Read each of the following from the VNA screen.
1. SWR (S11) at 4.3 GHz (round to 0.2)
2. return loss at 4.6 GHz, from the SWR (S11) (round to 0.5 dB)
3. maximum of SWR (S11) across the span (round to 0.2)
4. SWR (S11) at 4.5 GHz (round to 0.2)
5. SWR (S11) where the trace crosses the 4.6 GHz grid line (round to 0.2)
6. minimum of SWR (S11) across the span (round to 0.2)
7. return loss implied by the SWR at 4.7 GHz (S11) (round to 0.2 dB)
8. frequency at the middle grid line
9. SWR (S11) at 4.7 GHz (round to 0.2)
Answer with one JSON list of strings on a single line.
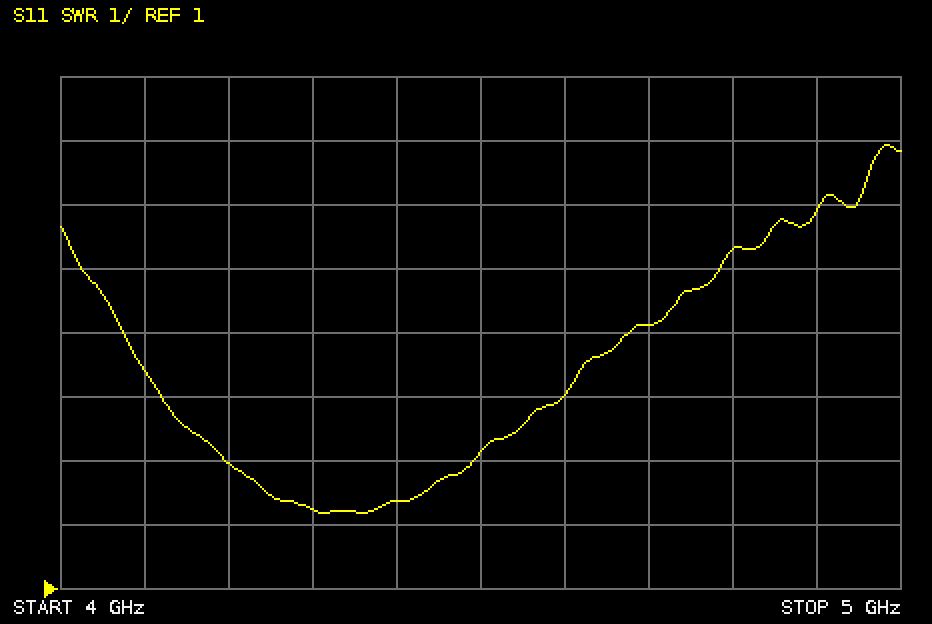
["2.2", "4.5 dB", "8.0", "3.2", "4.0", "2.2", "3.4 dB", "4.5 GHz", "5.2"]
